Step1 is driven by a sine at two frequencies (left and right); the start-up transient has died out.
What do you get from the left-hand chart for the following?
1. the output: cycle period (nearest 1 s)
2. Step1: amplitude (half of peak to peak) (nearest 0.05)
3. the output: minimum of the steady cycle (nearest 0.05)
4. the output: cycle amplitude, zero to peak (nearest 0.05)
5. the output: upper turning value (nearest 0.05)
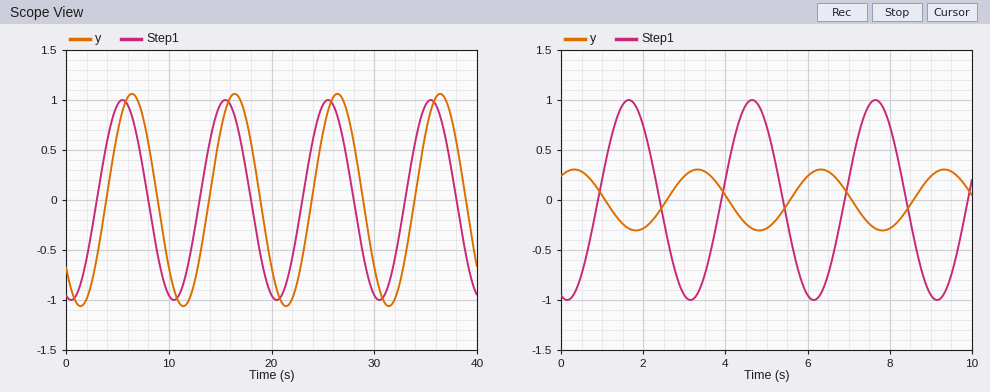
10 s
1.00
-1.05
1.05
1.05
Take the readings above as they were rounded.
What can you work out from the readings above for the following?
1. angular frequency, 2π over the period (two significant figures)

0.63 rad/s
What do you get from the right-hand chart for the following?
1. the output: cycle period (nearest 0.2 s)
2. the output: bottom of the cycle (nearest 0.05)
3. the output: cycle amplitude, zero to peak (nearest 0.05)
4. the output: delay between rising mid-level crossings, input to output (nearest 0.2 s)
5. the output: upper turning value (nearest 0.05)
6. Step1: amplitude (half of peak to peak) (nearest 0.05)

3.0 s
-0.30
0.30
1.6 s
0.30
1.00
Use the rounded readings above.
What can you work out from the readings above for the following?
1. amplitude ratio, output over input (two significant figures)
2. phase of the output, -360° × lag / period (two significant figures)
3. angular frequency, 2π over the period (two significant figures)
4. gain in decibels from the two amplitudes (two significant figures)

0.30
-190°
2.1 rad/s
-10 dB
